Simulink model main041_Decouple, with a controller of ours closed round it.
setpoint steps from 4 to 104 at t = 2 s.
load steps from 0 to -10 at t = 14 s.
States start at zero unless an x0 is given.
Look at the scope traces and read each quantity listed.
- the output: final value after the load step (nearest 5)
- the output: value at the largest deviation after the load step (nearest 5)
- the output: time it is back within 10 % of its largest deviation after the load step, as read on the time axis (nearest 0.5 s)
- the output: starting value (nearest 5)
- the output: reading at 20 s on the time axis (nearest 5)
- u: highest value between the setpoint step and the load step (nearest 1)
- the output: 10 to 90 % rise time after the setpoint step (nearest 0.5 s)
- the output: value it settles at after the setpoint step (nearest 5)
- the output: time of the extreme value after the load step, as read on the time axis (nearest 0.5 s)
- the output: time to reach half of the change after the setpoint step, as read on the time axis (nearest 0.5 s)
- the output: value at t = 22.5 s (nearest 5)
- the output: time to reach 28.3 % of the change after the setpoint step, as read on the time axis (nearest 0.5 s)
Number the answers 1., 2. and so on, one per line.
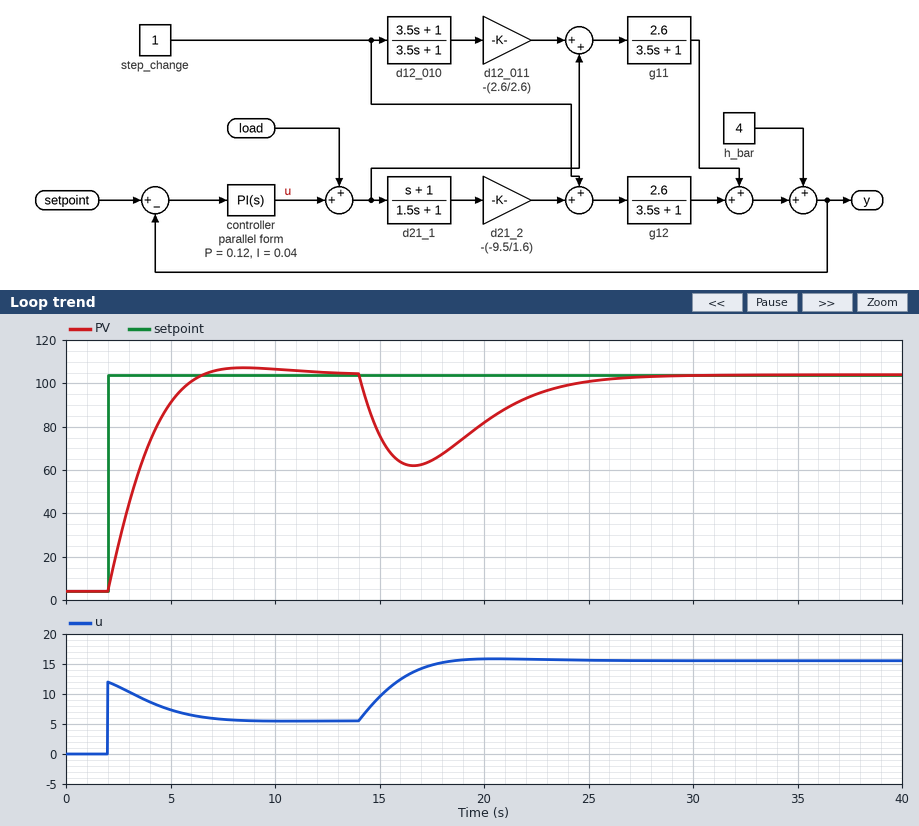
1. 105
2. 60
3. 24.5 s
4. 5
5. 80
6. 12
7. 3.0 s
8. 105
9. 16.5 s
10. 3.5 s
11. 95
12. 2.5 s
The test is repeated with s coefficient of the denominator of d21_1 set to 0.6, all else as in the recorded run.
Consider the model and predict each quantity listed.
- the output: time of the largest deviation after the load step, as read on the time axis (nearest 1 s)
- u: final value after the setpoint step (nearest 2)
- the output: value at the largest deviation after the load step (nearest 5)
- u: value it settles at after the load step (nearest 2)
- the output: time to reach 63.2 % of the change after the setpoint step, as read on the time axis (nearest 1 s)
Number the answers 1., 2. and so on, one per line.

1. 16 s
2. 6
3. 65
4. 16
5. 3 s
